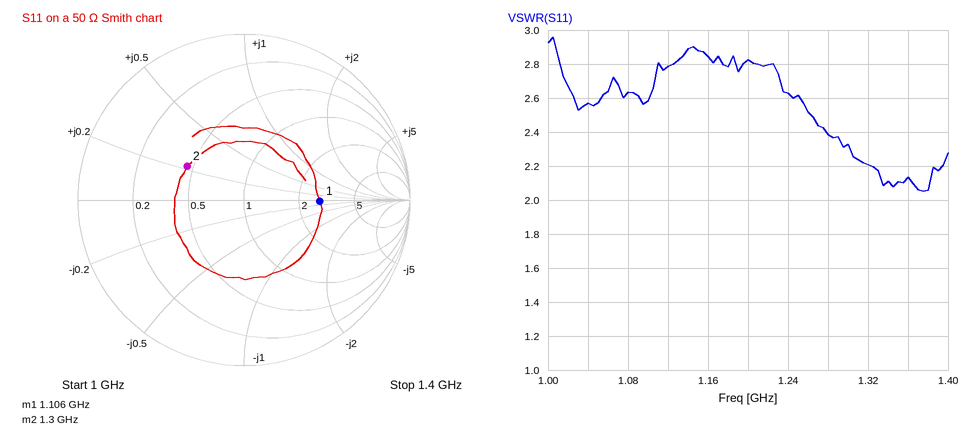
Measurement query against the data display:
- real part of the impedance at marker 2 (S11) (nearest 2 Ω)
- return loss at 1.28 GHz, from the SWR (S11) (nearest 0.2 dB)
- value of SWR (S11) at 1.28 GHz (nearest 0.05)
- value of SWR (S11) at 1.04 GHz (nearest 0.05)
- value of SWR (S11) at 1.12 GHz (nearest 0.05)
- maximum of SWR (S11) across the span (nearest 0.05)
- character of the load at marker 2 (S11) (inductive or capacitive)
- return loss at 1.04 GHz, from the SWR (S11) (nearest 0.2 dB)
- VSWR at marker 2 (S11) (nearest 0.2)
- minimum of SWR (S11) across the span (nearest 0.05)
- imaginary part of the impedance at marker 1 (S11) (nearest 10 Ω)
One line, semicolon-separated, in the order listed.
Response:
22 Ω; 7.8 dB; 2.40; 2.55; 2.80; 2.95; inductive; 7.2 dB; 2.4; 2.05; 0 Ω
